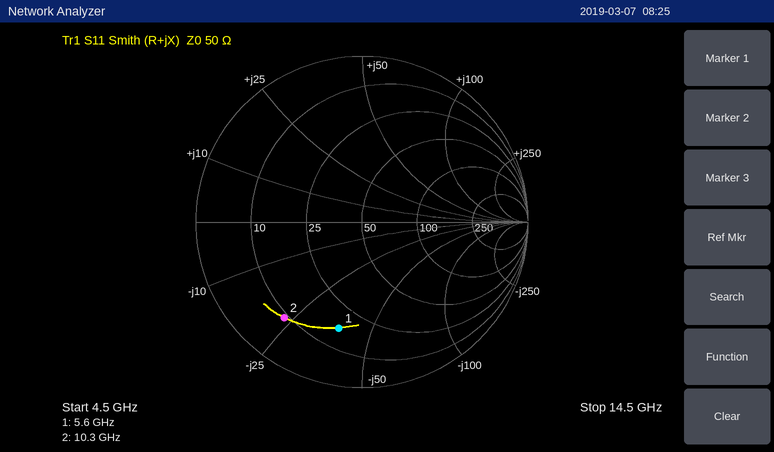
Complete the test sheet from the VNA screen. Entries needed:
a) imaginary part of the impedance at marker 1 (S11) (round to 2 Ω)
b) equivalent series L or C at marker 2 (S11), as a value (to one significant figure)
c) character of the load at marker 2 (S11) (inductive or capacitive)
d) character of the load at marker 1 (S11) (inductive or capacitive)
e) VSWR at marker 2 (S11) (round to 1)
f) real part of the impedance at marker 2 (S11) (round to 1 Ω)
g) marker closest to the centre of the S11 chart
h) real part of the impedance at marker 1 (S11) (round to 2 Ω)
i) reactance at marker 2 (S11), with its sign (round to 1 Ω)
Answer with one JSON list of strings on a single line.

["-38 Ω", "700 fF", "capacitive", "capacitive", "7", "9 Ω", "marker 1", "16 Ω", "-23 Ω"]
